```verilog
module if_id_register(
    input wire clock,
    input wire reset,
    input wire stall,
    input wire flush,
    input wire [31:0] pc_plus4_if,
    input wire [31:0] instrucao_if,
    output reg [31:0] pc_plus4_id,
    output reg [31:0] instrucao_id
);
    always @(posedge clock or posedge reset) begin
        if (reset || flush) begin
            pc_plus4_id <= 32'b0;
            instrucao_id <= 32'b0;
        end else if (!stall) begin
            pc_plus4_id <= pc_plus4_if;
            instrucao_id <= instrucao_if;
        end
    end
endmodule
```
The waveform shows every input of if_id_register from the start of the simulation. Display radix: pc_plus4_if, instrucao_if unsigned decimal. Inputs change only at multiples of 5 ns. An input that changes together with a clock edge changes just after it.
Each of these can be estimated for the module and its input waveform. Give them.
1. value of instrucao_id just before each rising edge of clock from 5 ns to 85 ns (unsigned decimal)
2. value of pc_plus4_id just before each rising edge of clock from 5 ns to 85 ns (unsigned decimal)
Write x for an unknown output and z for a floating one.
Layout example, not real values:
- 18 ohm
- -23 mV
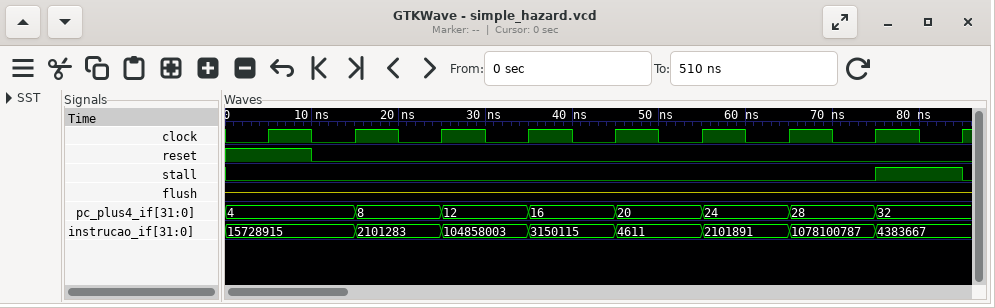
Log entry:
- 0, 0, 15728915, 2101283, 104858003, 3150115, 4611, 2101891, 1078100787
- 0, 0, 4, 8, 12, 16, 20, 24, 28
